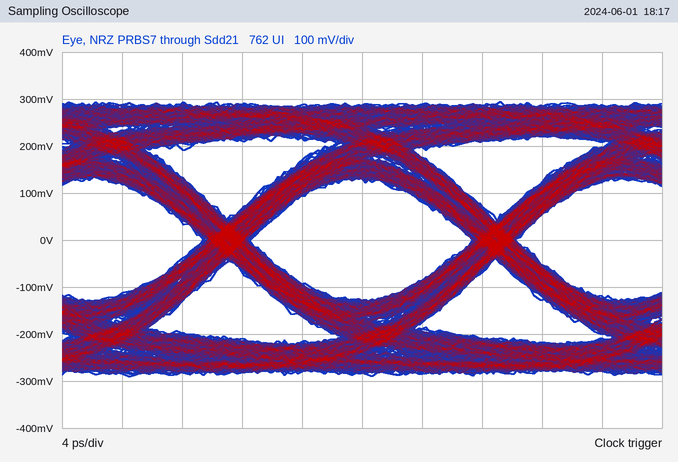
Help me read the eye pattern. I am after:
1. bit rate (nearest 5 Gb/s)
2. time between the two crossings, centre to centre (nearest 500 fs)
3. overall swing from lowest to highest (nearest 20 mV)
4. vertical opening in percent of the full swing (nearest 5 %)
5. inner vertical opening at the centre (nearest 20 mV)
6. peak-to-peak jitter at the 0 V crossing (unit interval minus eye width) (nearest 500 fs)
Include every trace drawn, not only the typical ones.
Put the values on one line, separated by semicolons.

55 Gb/s; 18.0 ps; 580 mV; 45 %; 260 mV; 3.0 ps
